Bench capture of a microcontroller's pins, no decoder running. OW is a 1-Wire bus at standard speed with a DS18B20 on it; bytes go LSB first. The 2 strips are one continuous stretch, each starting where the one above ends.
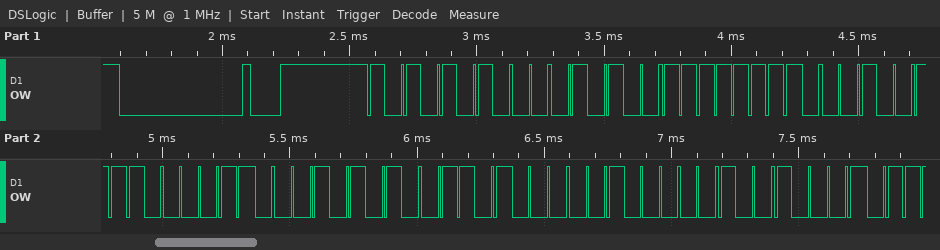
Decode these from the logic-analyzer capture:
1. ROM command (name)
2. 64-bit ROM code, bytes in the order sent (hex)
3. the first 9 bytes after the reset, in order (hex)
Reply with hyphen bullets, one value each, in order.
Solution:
- Match ROM
- 28 FF C8 61 54 16 04 89
- 55 28 FF C8 61 54 16 04 89
